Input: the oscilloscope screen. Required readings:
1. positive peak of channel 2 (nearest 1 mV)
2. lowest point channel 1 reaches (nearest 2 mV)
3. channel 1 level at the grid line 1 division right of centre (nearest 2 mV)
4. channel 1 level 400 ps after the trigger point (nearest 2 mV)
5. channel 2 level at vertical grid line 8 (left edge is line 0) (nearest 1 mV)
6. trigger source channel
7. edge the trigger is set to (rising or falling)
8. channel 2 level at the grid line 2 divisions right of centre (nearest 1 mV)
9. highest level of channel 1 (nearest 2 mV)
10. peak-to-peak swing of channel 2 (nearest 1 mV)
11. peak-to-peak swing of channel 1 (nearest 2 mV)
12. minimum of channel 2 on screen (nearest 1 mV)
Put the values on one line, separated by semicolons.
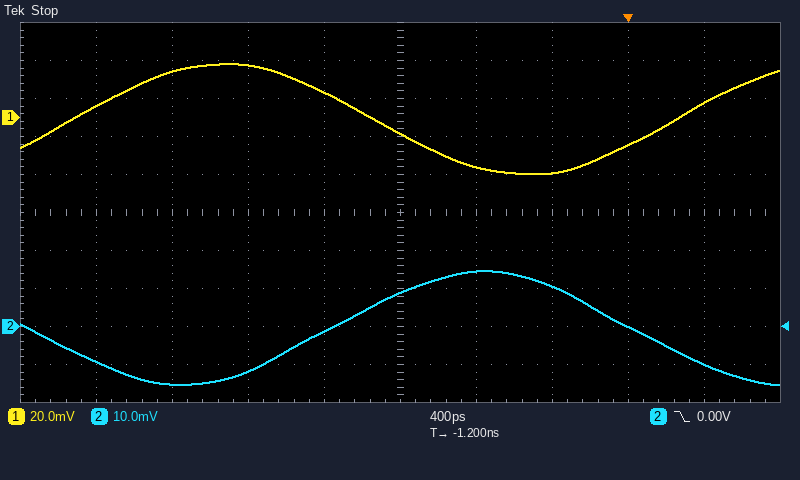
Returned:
15 mV; -30 mV; -26 mV; 8 mV; 0 mV; channel 2; falling; 11 mV; 28 mV; 30 mV; 58 mV; -15 mV
